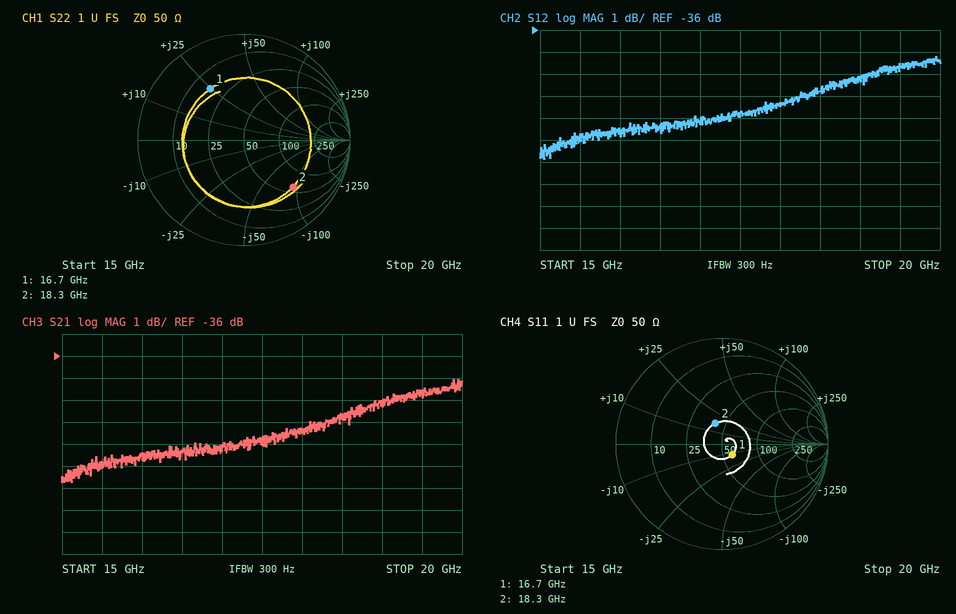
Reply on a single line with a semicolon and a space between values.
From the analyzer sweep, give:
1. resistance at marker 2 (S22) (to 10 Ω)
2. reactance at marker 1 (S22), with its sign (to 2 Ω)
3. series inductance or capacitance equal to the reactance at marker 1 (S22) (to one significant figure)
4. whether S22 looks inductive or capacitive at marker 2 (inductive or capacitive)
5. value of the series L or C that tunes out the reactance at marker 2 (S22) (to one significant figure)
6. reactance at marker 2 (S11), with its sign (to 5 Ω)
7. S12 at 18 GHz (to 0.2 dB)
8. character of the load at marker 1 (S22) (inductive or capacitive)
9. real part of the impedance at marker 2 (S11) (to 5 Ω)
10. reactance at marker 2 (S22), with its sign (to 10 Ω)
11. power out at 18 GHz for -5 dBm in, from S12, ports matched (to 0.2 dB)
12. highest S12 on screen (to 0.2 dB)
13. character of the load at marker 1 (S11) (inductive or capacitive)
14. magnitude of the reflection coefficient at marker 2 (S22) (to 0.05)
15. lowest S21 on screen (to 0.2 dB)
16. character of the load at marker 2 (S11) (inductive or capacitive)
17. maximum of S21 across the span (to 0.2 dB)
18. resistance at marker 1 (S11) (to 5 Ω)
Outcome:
60 Ω; +24 Ω; 200 pH; capacitive; 800 pH; +15 Ω; -39.4 dB; inductive; 40 Ω; -90 Ω; -44.4 dBm; -37.2 dB; capacitive; 0.65; -41.8 dB; inductive; -37.0 dB; 60 Ω
